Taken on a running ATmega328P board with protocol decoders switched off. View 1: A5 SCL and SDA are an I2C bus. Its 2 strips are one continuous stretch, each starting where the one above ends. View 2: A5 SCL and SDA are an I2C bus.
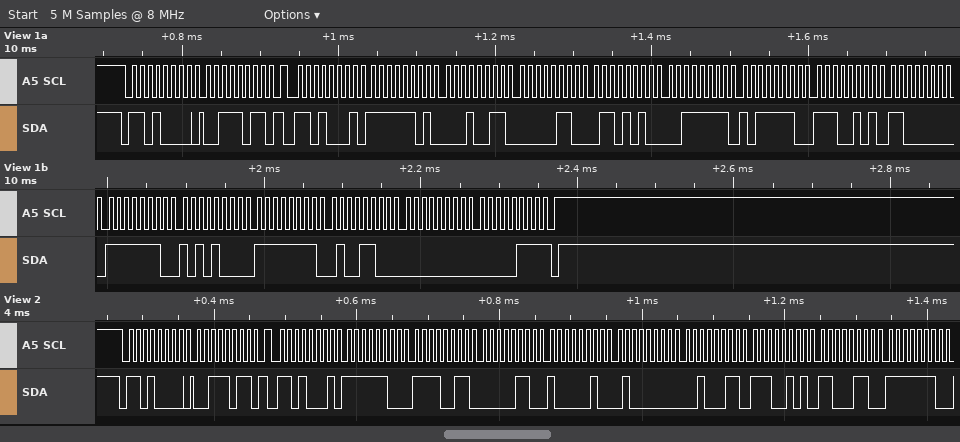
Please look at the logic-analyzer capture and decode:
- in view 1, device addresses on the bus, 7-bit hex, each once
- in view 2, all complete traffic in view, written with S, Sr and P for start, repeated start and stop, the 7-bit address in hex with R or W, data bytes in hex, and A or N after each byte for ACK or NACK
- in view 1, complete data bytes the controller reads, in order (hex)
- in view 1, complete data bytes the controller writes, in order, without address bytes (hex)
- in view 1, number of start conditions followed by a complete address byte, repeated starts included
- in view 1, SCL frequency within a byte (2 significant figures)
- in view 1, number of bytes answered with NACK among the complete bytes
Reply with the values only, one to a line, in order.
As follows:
0x68
S 68W A 3B A Sr 68R A FC A F3 A 06 A 82 A 40 A 23 A E5 A C6 A FE A
FD 13 06 6A 3F BE E5 C0 FE A8 FF 4C 00 07
3B
2
100 kHz
1
